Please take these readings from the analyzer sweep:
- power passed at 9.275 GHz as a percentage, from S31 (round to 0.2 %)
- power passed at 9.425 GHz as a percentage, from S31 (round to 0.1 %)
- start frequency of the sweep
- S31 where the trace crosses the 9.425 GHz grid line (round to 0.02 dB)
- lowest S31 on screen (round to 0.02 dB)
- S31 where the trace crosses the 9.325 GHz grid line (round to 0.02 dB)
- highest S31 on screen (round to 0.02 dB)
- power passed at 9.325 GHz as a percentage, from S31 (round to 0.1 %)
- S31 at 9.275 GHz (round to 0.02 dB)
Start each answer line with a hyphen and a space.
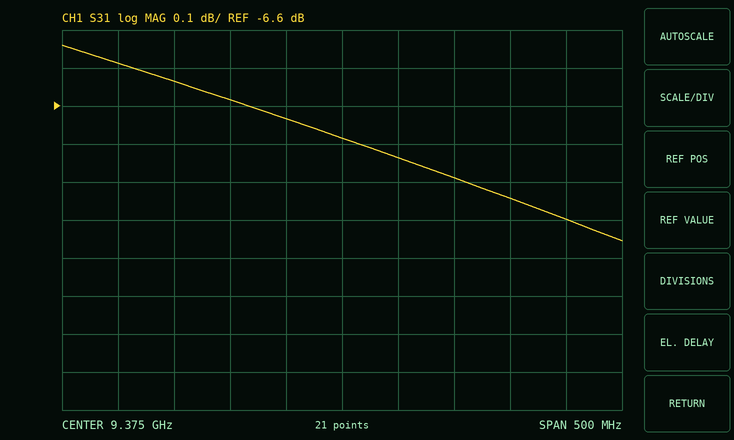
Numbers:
- 22.0 %
- 21.2 %
- 9.125 GHz
- -6.74 dB
- -6.96 dB
- -6.64 dB
- -6.44 dB
- 21.7 %
- -6.58 dB
